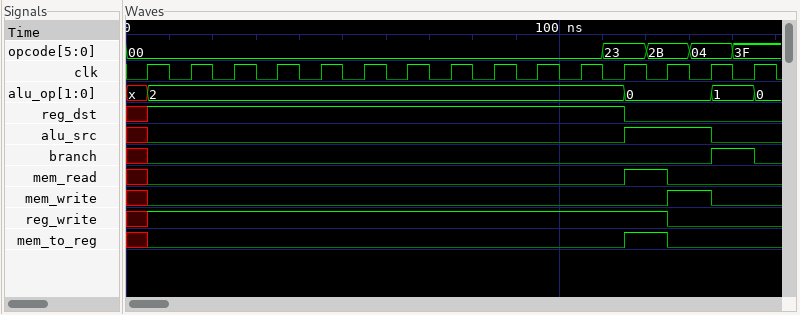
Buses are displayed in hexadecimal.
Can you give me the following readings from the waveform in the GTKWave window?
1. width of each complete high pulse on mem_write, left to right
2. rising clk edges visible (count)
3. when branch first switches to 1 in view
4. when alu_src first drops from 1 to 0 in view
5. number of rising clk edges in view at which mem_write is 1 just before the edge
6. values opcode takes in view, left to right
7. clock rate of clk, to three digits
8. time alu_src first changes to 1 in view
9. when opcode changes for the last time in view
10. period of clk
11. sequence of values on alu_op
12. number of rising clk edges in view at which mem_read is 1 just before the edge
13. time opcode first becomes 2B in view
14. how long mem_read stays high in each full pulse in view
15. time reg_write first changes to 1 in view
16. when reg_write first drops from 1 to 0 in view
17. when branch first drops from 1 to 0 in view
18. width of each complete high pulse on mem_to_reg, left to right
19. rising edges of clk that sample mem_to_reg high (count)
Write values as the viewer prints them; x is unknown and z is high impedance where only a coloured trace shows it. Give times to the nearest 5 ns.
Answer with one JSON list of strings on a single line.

["10 ns", "15", "135 ns", "135 ns", "1", "00, 23, 2B, 04, 3F", "100 MHz", "115 ns", "140 ns", "10 ns", "x, 2, 0, 1, 0", "1", "120 ns", "10 ns", "5 ns", "125 ns", "145 ns", "10 ns", "1"]
